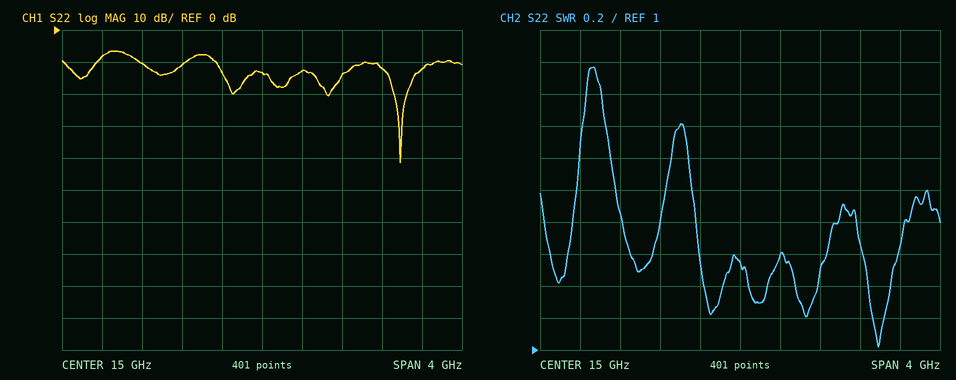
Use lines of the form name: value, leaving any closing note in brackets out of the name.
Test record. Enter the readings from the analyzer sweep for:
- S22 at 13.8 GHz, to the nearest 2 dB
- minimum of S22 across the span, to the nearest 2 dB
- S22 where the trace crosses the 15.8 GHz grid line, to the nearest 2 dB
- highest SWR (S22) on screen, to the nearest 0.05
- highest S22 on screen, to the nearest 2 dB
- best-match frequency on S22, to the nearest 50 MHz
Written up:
S22 at 13.8 GHz, to the nearest 2 dB: -10 dB
minimum of S22 across the span, to the nearest 2 dB: -42 dB
S22 where the trace crosses the 15.8 GHz grid line, to the nearest 2 dB: -14 dB
highest SWR (S22) on screen, to the nearest 0.05: 2.75
highest S22 on screen, to the nearest 2 dB: -6 dB
best-match frequency on S22, to the nearest 50 MHz: 16.40 GHz
